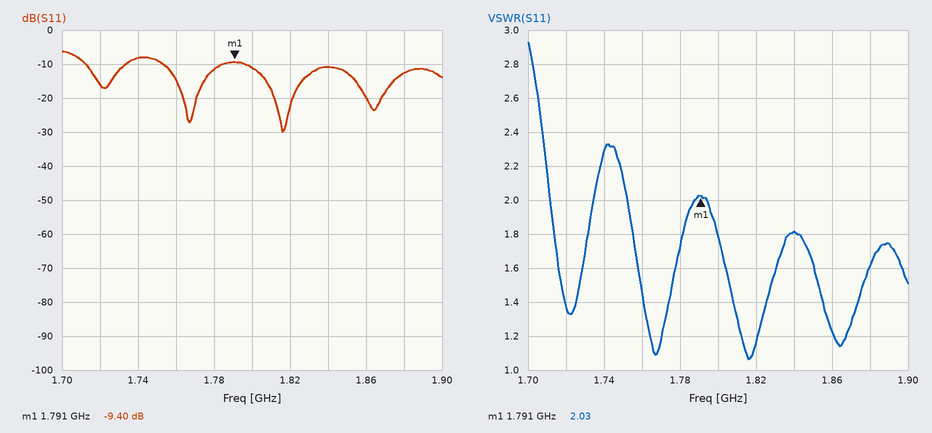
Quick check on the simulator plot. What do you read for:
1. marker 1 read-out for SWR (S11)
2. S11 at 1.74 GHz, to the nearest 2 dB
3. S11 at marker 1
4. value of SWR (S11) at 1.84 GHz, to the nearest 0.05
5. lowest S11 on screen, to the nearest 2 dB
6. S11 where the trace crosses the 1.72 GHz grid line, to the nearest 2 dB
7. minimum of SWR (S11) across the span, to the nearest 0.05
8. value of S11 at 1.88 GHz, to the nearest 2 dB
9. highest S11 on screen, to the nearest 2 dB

2.03
-8 dB
-9.40 dB
1.80
-30 dB
-16 dB
1.05
-12 dB
-6 dB
